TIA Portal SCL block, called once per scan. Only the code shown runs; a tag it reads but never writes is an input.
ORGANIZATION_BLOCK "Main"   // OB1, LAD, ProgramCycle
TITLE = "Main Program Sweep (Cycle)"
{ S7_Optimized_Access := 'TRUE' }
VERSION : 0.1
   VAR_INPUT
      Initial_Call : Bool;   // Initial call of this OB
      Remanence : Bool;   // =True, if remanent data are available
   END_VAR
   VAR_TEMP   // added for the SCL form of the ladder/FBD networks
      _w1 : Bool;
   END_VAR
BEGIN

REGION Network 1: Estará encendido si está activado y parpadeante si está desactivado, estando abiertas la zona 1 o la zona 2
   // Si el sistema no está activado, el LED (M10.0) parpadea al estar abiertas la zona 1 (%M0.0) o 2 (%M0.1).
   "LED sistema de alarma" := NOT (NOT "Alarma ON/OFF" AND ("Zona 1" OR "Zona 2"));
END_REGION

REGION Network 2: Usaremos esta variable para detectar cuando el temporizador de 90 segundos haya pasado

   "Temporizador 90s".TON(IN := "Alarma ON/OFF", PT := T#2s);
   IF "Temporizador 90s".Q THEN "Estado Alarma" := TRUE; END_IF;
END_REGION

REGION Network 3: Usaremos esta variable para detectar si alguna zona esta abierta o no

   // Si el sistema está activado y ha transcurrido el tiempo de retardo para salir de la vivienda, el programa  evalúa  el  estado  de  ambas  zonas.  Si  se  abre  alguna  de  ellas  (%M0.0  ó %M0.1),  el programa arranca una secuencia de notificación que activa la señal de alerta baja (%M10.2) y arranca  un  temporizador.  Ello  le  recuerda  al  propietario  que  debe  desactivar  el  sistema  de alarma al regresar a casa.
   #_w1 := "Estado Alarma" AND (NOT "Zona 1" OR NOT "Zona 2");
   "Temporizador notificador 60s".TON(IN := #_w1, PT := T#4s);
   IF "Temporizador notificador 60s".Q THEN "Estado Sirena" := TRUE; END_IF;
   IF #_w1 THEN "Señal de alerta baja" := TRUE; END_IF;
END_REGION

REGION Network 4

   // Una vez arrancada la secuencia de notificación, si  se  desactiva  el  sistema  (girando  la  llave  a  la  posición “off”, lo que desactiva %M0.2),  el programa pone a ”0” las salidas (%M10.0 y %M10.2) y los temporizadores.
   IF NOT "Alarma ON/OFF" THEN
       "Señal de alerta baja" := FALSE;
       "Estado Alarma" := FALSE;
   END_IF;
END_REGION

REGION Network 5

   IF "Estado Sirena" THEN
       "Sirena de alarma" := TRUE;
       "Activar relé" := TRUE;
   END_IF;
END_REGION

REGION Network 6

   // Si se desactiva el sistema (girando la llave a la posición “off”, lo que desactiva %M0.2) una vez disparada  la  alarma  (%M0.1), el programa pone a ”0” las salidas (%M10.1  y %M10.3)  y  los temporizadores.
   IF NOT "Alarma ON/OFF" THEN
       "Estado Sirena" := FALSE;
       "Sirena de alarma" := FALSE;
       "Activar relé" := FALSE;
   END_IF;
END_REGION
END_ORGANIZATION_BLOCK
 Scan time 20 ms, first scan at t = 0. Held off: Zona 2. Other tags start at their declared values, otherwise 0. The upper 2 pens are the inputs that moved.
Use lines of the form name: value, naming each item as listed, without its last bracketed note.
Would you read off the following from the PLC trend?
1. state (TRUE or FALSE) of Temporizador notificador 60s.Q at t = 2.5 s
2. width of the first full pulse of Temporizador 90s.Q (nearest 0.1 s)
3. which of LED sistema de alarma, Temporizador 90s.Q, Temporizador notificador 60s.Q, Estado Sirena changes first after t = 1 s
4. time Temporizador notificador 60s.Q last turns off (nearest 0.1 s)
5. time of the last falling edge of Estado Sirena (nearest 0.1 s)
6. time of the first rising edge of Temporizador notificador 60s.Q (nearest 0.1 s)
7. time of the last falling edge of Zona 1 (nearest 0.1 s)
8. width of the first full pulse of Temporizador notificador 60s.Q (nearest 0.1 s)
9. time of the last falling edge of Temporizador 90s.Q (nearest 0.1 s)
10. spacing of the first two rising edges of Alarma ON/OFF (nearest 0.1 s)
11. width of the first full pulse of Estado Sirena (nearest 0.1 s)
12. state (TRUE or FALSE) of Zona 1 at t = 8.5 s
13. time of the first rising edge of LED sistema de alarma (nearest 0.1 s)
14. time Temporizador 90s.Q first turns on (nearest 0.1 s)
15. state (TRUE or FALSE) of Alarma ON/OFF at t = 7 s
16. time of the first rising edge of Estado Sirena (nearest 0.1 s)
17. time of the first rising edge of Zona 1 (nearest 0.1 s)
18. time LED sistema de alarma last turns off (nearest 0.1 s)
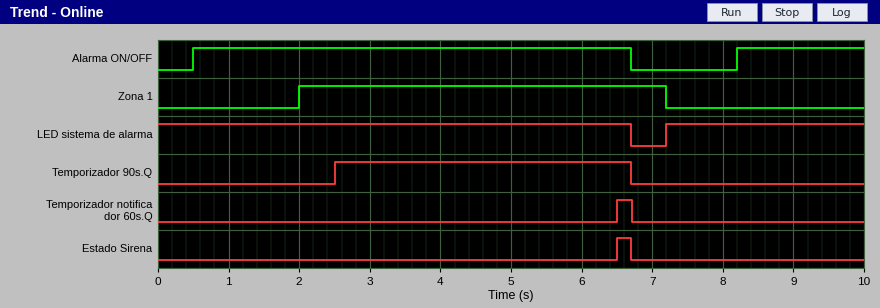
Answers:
state (TRUE or FALSE) of Temporizador notificador 60s.Q at t = 2.5 s: FALSE
width of the first full pulse of Temporizador 90s.Q: 4.2 s
which of LED sistema de alarma, Temporizador 90s.Q, Temporizador notificador 60s.Q, Estado Sirena changes first after t = 1 s: Temporizador 90s.Q
time Temporizador notificador 60s.Q last turns off: 6.7 s
time of the last falling edge of Estado Sirena: 6.7 s
time of the first rising edge of Temporizador notificador 60s.Q: 6.5 s
time of the last falling edge of Zona 1: 7.2 s
width of the first full pulse of Temporizador notificador 60s.Q: 0.2 s
time of the last falling edge of Temporizador 90s.Q: 6.7 s
spacing of the first two rising edges of Alarma ON/OFF: 7.7 s
width of the first full pulse of Estado Sirena: 0.2 s
state (TRUE or FALSE) of Zona 1 at t = 8.5 s: FALSE
time of the first rising edge of LED sistema de alarma: 7.2 s
time Temporizador 90s.Q first turns on: 2.5 s
state (TRUE or FALSE) of Alarma ON/OFF at t = 7 s: FALSE
time of the first rising edge of Estado Sirena: 6.5 s
time of the first rising edge of Zona 1: 2.0 s
time LED sistema de alarma last turns off: 6.7 s
